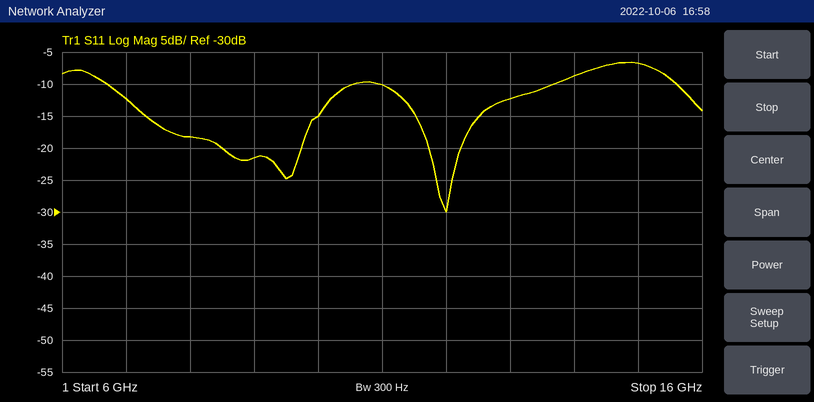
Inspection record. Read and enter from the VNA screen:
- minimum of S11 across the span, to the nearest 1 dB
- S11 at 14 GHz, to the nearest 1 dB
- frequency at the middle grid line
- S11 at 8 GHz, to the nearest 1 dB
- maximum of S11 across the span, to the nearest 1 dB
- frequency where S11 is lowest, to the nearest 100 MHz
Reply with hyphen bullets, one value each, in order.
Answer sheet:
- -30 dB
- -9 dB
- 11 GHz
- -18 dB
- -7 dB
- 12.0 GHz
